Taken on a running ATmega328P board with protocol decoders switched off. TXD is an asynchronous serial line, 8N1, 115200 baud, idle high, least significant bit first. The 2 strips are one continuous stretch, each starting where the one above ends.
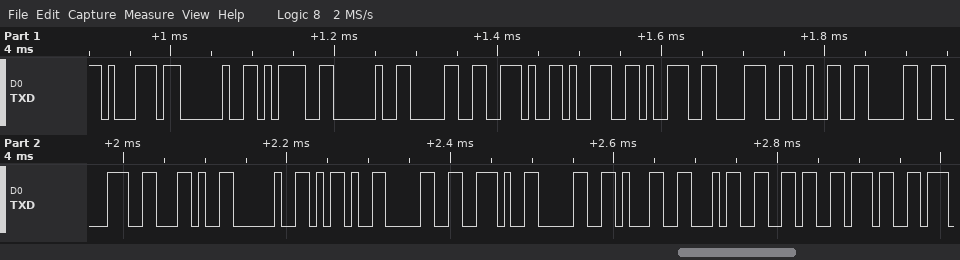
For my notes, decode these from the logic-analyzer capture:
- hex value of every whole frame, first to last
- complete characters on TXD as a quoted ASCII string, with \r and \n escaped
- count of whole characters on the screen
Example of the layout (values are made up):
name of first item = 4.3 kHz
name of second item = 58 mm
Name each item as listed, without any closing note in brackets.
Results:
hex value of every whole frame, first to last = 0x71 0x20 0x3D 0x20 0x30 0x2E 0x39 0x39 0x38 0x32 0x30 0x38 0x2C 0x20 0x2D 0x30 0x2E 0x30 0x31 0x34 0x36 0x37
complete characters on TXD as a quoted ASCII string, with \r and \n escaped = "q = 0.998208, -0.01467"
count of whole characters on the screen = 22
